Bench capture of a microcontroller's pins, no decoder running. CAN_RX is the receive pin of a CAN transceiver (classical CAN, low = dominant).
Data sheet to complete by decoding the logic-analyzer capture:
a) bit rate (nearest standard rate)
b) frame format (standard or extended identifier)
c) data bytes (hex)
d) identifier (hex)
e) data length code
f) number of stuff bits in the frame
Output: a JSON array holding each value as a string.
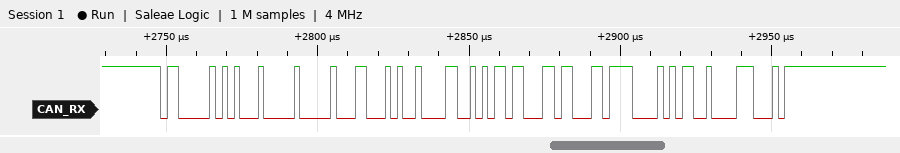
["500 kbit/s", "standard", "00 31 48 65 6C 6C 6F 0A", "0x605", "8", "3"]
